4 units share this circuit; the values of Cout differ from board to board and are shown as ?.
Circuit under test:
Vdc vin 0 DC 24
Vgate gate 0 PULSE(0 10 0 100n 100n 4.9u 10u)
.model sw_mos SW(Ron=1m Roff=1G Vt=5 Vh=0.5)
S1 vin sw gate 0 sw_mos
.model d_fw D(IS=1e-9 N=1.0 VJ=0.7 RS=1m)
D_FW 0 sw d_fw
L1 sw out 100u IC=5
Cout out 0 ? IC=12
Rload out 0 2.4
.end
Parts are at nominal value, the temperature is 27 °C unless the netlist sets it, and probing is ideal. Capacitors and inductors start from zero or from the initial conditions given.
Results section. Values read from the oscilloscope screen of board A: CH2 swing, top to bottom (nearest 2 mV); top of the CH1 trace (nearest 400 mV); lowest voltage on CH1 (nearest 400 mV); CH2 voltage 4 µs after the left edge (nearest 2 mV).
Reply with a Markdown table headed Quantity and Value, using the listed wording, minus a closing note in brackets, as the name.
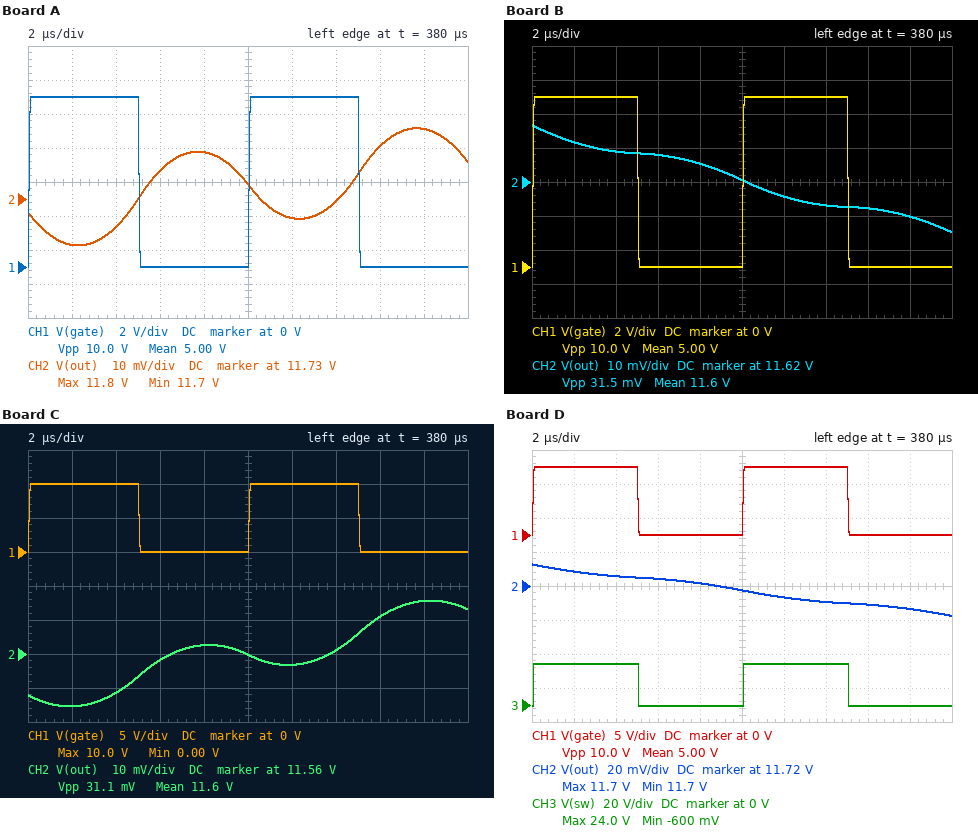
| Quantity | Value |
|---|---|
| CH2 swing, top to bottom | 34 mV |
| top of the CH1 trace | 10.0 V |
| lowest voltage on CH1 | 0 V |
| CH2 voltage 4 µs after the left edge | 11.722 V |
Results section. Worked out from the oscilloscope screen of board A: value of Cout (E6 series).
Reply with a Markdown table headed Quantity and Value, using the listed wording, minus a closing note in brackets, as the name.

| Quantity | Value |
|---|---|
| value of Cout | 33 µF |
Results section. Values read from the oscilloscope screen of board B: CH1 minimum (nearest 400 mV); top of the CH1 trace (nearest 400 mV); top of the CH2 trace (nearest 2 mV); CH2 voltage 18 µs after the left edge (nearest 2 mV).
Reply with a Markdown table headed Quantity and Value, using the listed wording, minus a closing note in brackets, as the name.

| Quantity | Value |
|---|---|
| CH1 minimum | 0 V |
| top of the CH1 trace | 10.0 V |
| top of the CH2 trace | 11.636 V |
| CH2 voltage 18 µs after the left edge | 11.610 V |
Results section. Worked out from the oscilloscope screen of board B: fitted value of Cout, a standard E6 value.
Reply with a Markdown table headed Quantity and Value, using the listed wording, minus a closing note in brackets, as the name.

| Quantity | Value |
|---|---|
| fitted value of Cout, a standard E6 value | 220 µF |
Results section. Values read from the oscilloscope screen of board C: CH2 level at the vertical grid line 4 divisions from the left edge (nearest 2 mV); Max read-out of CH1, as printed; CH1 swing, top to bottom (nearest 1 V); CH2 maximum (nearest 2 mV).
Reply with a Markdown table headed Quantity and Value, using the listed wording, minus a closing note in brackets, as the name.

| Quantity | Value |
|---|---|
| CH2 level at the vertical grid line 4 divisions from the left edge | 11.562 V |
| Max read-out of CH1, as printed | 10.0 V |
| CH1 swing, top to bottom | 10 V |
| CH2 maximum | 11.576 V |
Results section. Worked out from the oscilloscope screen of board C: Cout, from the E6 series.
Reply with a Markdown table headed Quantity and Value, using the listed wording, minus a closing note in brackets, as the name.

| Quantity | Value |
|---|---|
| Cout, from the E6 series | 68 µF |
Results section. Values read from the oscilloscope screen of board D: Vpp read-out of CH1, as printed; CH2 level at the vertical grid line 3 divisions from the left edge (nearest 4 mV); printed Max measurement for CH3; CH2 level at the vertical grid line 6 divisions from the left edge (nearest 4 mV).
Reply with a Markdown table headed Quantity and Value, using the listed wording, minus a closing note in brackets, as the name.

| Quantity | Value |
|---|---|
| Vpp read-out of CH1, as printed | 10.0 V |
| CH2 level at the vertical grid line 3 divisions from the left edge | 11.724 V |
| printed Max measurement for CH3 | 24.0 V |
| CH2 level at the vertical grid line 6 divisions from the left edge | 11.712 V |
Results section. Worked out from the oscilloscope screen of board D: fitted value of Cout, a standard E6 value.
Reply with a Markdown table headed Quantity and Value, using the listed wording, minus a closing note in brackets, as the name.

| Quantity | Value |
|---|---|
| fitted value of Cout, a standard E6 value | 330 µF |
